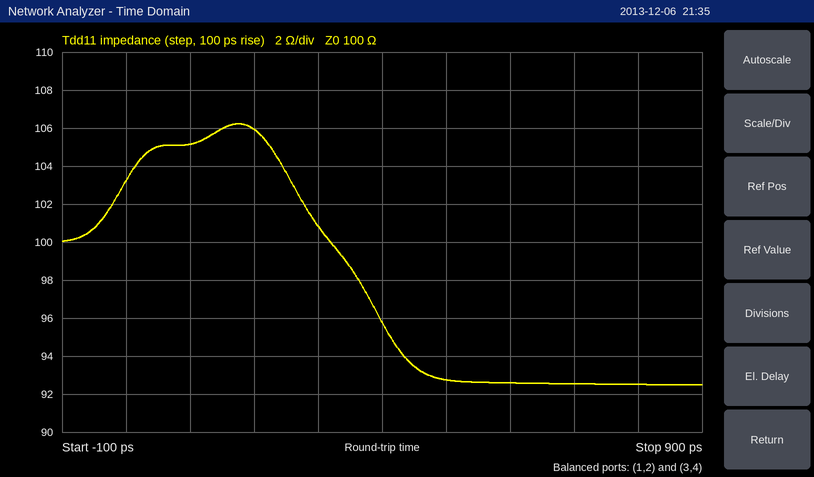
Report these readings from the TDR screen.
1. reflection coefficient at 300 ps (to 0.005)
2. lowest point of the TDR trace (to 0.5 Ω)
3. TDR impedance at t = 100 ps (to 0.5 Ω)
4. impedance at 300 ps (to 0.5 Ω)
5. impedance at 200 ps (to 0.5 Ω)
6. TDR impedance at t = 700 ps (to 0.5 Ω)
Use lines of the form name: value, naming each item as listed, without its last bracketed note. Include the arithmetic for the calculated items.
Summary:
reflection coefficient at 300 ps: (101 − 100)/(101 + 100) ≈ +0.005
lowest point of the TDR trace: 92.5 Ω
TDR impedance at t = 100 ps: 105.0 Ω
impedance at 300 ps: 101.0 Ω
impedance at 200 ps: 106.0 Ω
TDR impedance at t = 700 ps: 92.5 Ω
